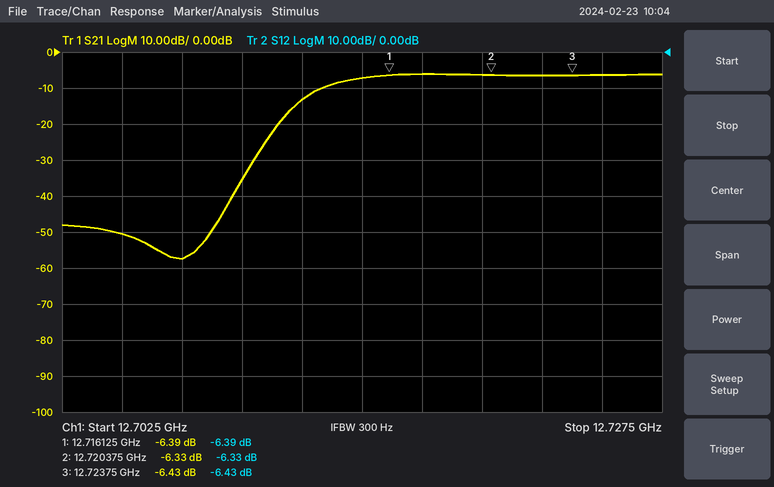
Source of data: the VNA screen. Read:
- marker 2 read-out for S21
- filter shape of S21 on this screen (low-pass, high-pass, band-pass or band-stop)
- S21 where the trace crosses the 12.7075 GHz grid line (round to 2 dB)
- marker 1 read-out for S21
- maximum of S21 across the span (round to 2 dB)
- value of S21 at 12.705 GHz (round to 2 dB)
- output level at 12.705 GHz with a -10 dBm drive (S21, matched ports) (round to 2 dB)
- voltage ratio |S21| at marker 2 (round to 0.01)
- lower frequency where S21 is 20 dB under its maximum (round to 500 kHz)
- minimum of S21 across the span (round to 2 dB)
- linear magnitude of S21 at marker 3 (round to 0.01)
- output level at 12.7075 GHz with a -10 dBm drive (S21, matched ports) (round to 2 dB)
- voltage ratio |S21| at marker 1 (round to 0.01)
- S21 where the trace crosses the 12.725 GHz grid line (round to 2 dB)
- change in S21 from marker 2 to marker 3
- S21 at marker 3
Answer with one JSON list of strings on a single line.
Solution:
["-6.33 dB", "high-pass", "-58 dB", "-6.39 dB", "-6 dB", "-50 dB", "-60 dBm", "0.48", "12.7110 GHz", "-58 dB", "0.48", "-68 dBm", "0.48", "-6 dB", "-0.10 dB", "-6.43 dB"]
